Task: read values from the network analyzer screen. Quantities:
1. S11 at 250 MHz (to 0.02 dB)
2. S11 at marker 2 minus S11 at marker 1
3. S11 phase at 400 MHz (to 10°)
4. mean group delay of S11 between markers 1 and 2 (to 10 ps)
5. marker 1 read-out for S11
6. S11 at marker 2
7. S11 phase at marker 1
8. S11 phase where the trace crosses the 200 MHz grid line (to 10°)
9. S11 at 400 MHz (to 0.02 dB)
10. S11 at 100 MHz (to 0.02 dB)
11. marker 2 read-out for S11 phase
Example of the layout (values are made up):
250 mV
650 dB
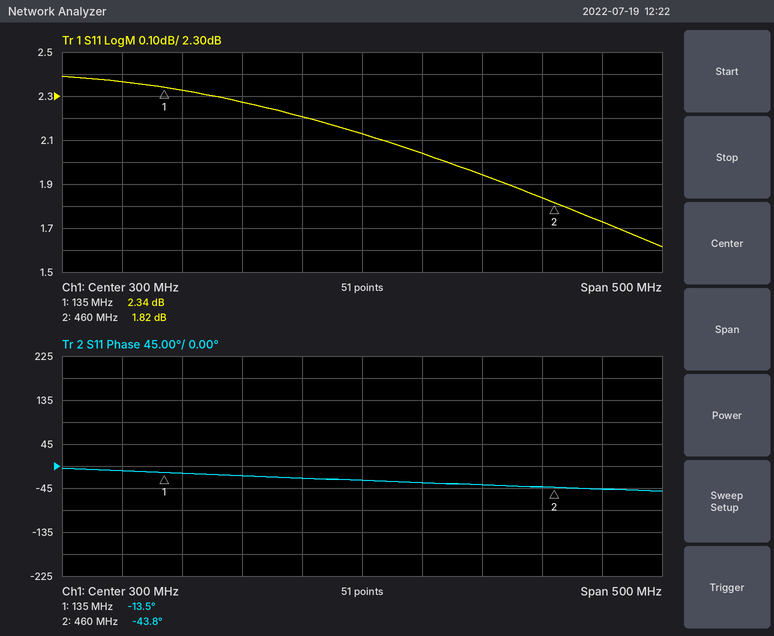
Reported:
2.20 dB
-0.52 dB
-40°
260 ps
2.34 dB
1.82 dB
-13.5°
-20°
1.94 dB
2.36 dB
-43.8°
